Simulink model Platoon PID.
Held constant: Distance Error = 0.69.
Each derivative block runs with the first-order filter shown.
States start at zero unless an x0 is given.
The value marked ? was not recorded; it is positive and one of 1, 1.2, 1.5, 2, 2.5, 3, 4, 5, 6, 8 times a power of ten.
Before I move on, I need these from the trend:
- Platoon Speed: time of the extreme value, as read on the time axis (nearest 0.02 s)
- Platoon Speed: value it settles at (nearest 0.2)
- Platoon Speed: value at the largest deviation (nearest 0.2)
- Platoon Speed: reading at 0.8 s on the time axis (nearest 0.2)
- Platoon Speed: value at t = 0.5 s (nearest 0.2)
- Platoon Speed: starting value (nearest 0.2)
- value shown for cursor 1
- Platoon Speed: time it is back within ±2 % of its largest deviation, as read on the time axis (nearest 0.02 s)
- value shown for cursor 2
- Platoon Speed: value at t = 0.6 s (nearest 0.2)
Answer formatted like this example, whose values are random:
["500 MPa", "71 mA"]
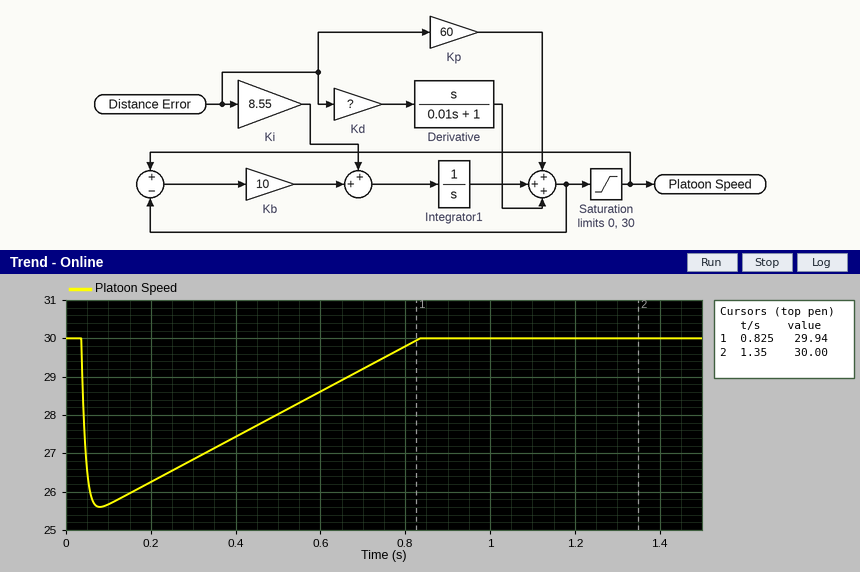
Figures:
["0.08 s", "30.0", "25.6", "29.8", "28.0", "30.0", "29.94", "0.82 s", "30.00", "28.6"]
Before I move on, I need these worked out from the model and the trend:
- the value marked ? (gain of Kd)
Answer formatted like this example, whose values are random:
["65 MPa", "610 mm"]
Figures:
["2.5"]
